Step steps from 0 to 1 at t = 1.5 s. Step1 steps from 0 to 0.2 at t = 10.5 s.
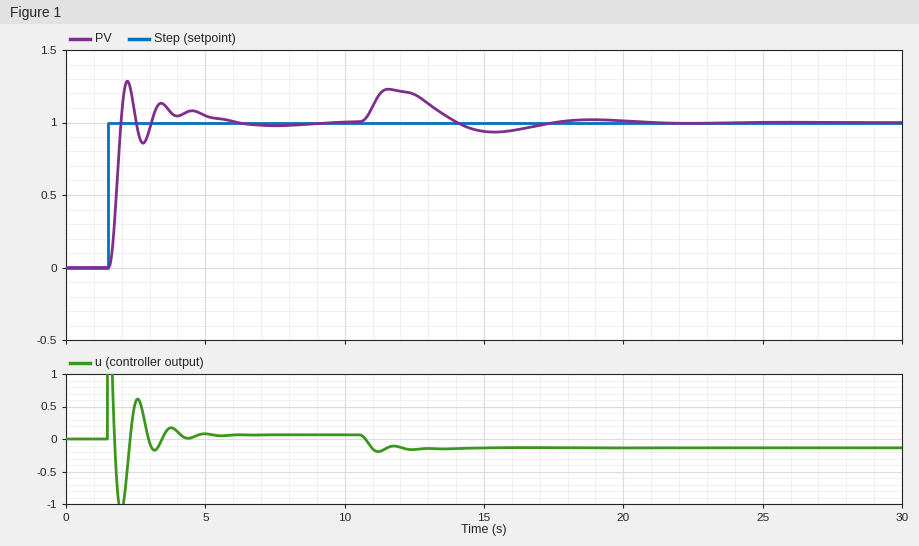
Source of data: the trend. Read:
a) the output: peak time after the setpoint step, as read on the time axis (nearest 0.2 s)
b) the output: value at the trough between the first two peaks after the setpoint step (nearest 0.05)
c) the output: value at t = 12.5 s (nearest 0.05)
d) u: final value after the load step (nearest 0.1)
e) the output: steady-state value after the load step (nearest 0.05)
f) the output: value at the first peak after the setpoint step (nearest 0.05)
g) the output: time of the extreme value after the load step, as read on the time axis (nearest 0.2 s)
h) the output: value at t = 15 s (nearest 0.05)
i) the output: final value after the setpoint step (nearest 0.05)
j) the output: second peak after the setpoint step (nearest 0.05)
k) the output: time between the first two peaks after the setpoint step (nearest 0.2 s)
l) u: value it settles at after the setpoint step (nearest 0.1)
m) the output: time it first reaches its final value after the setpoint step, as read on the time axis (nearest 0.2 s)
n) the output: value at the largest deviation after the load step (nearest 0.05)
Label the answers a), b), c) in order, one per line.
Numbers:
a) 2.2 s
b) 0.85
c) 1.20
d) -0.1
e) 1.00
f) 1.30
g) 11.6 s
h) 0.95
i) 1.00
j) 1.15
k) 1.2 s
l) 0.1
m) 2.0 s
n) 1.25
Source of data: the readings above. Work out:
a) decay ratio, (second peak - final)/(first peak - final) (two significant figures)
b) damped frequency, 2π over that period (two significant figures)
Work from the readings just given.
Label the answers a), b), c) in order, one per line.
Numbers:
a) 0.50
b) 5.2 rad/s
